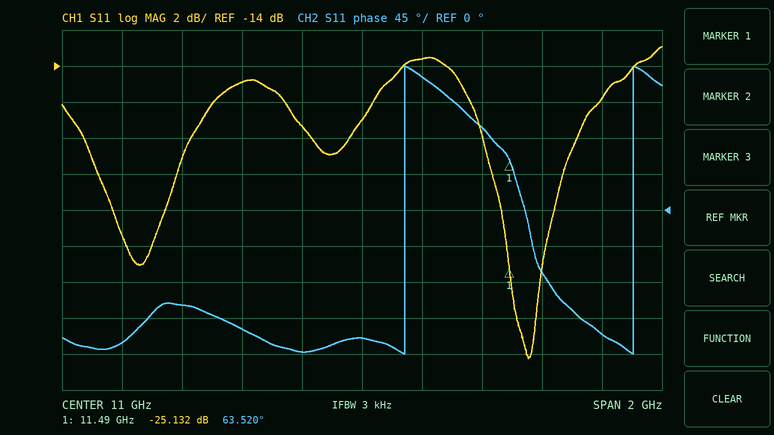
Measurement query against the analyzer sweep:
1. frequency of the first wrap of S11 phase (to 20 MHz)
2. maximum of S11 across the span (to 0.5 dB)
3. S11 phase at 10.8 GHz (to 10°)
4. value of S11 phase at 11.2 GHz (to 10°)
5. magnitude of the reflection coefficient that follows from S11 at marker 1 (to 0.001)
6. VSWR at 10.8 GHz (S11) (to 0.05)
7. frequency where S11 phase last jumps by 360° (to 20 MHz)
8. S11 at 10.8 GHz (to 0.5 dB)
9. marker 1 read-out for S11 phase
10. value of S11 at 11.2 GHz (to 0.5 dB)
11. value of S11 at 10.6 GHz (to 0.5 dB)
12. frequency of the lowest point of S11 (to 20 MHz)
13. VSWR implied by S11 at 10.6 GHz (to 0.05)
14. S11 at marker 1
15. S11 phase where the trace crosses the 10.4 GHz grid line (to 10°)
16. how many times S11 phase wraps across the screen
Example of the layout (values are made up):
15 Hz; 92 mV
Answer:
11.14 GHz; -13.0 dB; -180°; 170°; 0.055; 1.30; 11.90 GHz; -17.5 dB; 63.520°; -13.5 dB; -15.0 dB; 11.56 GHz; 1.45; -25.132 dB; -120°; 2
